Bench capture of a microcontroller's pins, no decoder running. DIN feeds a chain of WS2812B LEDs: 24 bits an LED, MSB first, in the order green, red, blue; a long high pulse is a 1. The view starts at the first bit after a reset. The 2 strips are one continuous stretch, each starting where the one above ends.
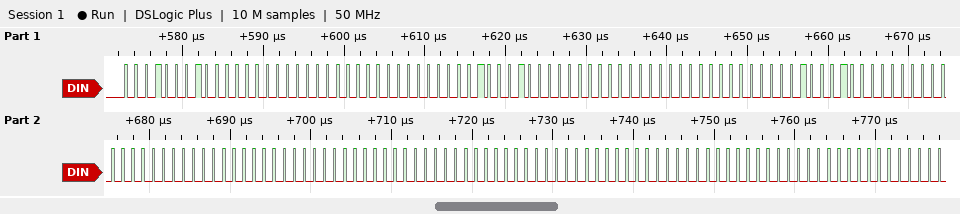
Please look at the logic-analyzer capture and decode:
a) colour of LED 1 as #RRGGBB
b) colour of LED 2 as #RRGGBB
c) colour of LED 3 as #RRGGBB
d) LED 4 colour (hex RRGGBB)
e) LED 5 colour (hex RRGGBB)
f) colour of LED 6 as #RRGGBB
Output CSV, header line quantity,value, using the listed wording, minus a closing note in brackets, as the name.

quantity,value
colour of LED 1 as #RRGGBB,#001100
colour of LED 2 as #RRGGBB,#110000
colour of LED 3 as #RRGGBB,#000011
LED 4 colour,#000000
LED 5 colour,#000000
colour of LED 6 as #RRGGBB,#000000
